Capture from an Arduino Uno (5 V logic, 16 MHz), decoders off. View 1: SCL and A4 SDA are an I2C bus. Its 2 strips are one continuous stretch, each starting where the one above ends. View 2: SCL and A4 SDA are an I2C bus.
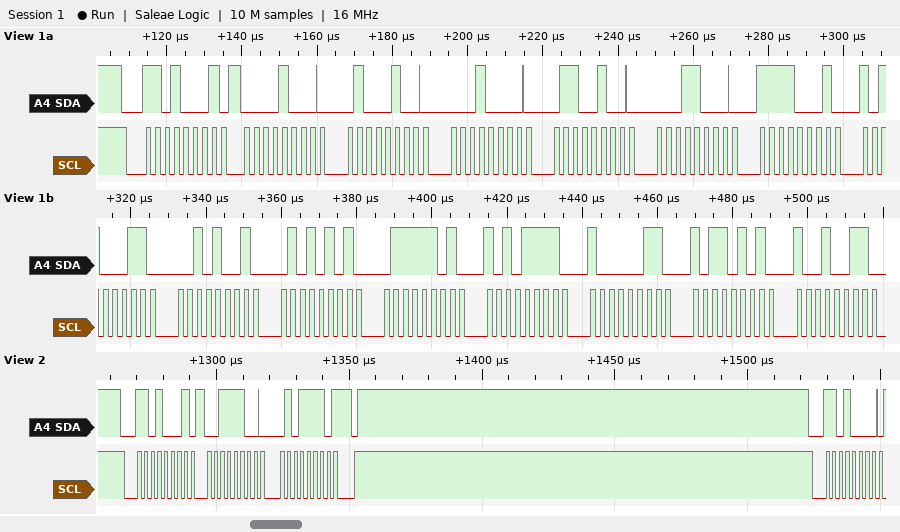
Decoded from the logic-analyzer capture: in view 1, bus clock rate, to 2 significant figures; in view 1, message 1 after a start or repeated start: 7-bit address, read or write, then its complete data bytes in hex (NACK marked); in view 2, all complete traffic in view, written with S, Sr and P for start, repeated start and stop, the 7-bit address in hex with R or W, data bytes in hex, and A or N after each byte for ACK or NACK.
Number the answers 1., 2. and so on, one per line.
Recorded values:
1. 400 kHz
2. 0x68 read: 08 44 10 64 18 F1 A3 29 55 7D AF 83 B5 93
3. S 68R A 3C A 5E N P S 68W A
